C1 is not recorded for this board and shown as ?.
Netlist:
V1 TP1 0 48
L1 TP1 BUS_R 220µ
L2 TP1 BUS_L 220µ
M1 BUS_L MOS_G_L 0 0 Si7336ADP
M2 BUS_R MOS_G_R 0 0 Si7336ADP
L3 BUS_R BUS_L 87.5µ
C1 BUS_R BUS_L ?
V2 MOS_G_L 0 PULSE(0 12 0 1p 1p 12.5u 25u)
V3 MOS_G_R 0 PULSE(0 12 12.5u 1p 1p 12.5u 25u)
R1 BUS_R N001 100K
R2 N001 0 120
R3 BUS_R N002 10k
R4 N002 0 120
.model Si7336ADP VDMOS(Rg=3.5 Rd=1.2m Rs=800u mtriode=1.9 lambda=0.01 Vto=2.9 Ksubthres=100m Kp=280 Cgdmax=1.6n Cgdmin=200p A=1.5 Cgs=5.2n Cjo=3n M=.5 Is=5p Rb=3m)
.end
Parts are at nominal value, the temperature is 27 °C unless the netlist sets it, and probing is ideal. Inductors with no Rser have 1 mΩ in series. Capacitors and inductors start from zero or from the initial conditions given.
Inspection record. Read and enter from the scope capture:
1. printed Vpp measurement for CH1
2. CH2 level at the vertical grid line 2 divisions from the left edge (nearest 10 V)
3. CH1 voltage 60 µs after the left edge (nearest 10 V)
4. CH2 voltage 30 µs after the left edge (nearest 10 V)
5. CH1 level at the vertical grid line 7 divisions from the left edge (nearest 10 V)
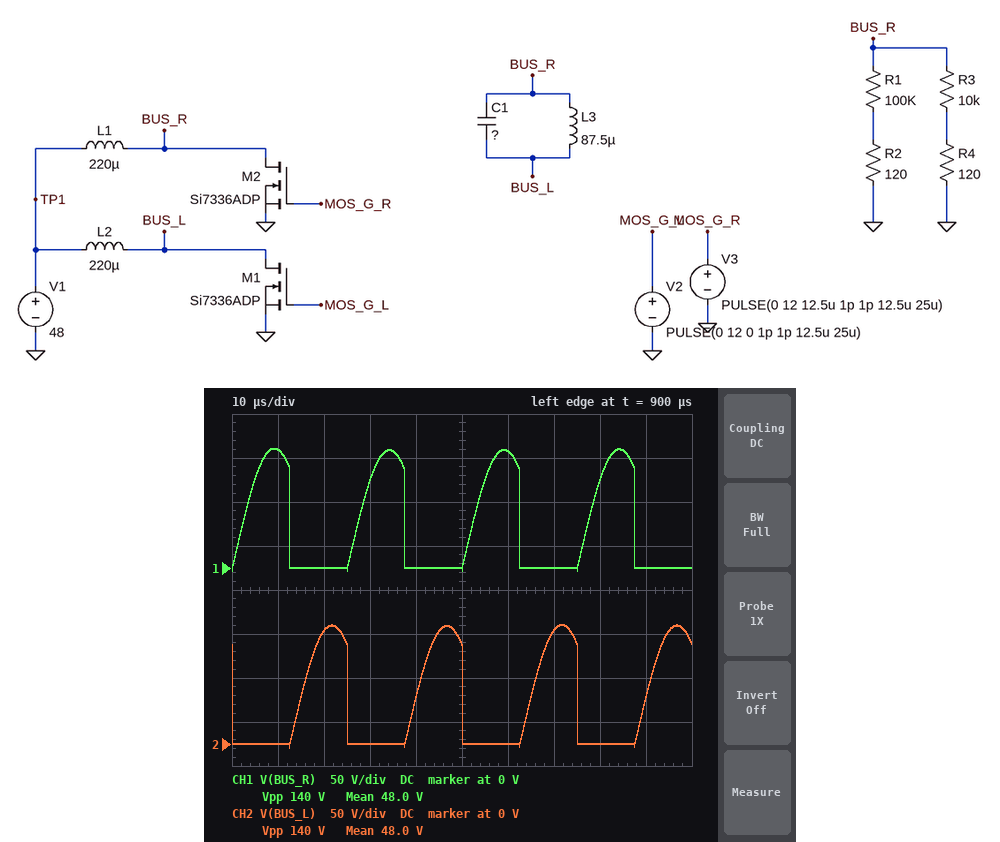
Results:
140 V
130 V
130 V
0 V
0 V
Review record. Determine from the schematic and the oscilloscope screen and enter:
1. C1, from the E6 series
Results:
470 nF
